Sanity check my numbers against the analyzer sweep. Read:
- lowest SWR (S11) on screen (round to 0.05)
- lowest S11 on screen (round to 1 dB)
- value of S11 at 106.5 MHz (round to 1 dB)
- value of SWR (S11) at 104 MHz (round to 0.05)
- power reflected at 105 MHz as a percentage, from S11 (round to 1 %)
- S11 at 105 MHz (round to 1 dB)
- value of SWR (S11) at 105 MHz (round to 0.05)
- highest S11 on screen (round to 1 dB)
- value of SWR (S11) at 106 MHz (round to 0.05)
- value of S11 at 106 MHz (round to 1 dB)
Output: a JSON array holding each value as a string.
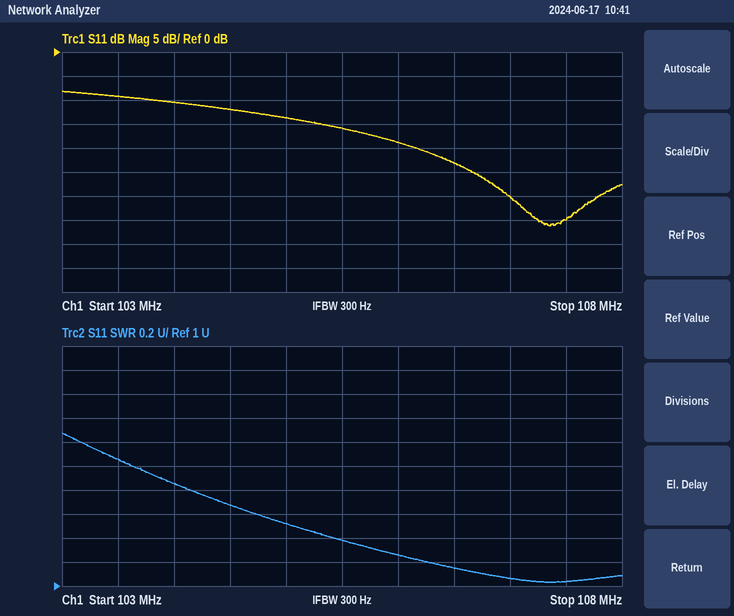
["1.05", "-36 dB", "-23 dB", "1.85", "4 %", "-14 dB", "1.50", "-8 dB", "1.25", "-19 dB"]
